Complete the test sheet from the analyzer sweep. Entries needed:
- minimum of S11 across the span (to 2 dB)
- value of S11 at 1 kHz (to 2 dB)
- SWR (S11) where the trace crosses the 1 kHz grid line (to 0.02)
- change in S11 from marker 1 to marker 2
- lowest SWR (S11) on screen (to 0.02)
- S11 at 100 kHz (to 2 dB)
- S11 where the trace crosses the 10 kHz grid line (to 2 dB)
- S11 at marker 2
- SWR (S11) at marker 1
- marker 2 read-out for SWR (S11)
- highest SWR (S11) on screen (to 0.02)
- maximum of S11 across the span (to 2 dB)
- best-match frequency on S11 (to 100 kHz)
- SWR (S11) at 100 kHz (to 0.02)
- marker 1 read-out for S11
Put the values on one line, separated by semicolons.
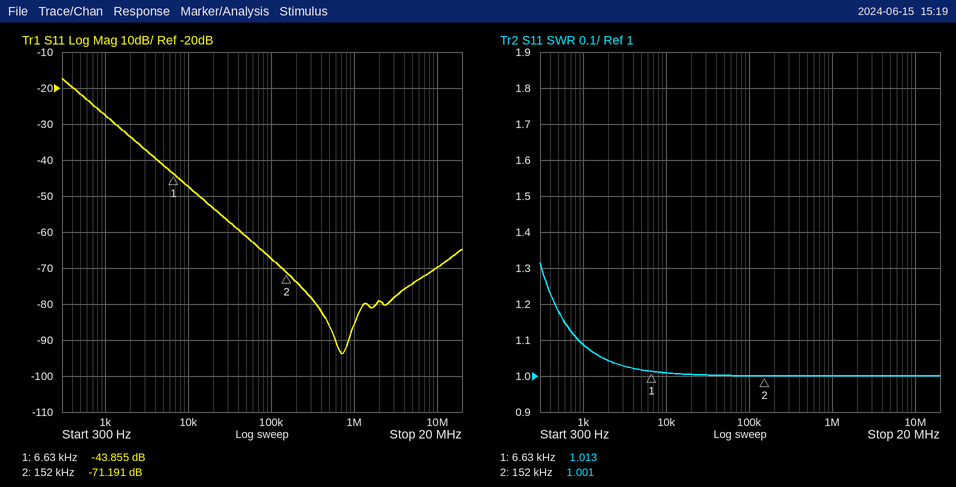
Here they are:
-94 dB; -28 dB; 1.08; -27.336 dB; 1.00; -68 dB; -48 dB; -71.191 dB; 1.013; 1.001; 1.32; -18 dB; 700 kHz; 1.00; -43.855 dB
